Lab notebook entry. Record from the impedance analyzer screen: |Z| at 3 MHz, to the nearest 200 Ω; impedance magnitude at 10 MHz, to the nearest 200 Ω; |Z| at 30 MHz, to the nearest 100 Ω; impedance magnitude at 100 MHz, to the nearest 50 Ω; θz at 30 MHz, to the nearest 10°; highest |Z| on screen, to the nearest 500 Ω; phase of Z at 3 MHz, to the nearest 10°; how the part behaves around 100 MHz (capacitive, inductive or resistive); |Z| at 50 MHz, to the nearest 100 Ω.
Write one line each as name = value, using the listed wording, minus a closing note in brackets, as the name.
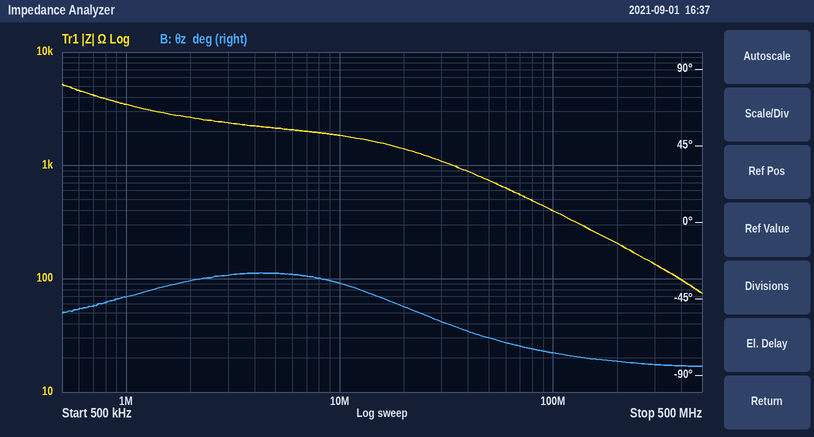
|Z| at 3 MHz, to the nearest 200 Ω = 2.4 kΩ
impedance magnitude at 10 MHz, to the nearest 200 Ω = 1.8 kΩ
|Z| at 30 MHz, to the nearest 100 Ω = 1.1 kΩ
impedance magnitude at 100 MHz, to the nearest 50 Ω = 400 Ω
θz at 30 MHz, to the nearest 10° = -60°
highest |Z| on screen, to the nearest 500 Ω = 5.0 kΩ
phase of Z at 3 MHz, to the nearest 10° = -30°
how the part behaves around 100 MHz = capacitive
|Z| at 50 MHz, to the nearest 100 Ω = 700 Ω
